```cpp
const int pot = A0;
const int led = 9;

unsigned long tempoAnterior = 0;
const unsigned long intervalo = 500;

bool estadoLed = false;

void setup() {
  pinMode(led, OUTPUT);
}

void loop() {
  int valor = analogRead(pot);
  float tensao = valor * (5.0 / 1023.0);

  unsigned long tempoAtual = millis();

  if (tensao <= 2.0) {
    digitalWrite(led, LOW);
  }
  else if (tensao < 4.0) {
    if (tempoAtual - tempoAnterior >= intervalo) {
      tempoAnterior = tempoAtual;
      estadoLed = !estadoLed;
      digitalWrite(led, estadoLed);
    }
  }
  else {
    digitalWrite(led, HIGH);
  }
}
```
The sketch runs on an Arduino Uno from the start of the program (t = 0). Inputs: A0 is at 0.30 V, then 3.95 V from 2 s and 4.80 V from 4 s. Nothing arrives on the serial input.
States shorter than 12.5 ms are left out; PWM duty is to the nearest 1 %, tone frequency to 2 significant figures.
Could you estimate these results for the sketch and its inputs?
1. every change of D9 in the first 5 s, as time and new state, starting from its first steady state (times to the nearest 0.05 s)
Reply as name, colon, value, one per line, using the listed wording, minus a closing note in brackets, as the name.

every change of D9 in the first 5 s, as time and new state, starting from its first steady state: 0 s low; 2 s high; 2.5 s low; 3 s high; 3.5 s low; 4 s high
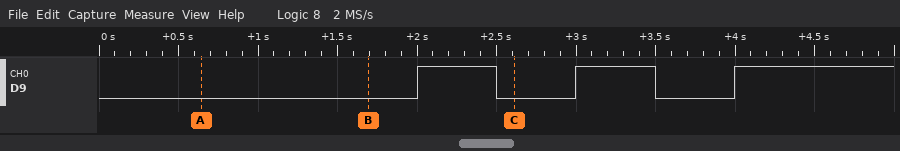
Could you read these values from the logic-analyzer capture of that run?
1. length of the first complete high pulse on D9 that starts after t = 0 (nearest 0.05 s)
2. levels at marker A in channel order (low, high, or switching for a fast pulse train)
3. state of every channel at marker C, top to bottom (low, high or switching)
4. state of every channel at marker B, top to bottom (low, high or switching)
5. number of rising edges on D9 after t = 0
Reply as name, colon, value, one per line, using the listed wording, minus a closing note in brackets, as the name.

length of the first complete high pulse on D9 that starts after t = 0: 0.50 s
levels at marker A in channel order: D9 low
state of every channel at marker C, top to bottom: D9 low
state of every channel at marker B, top to bottom: D9 low
number of rising edges on D9 after t = 0: 3
